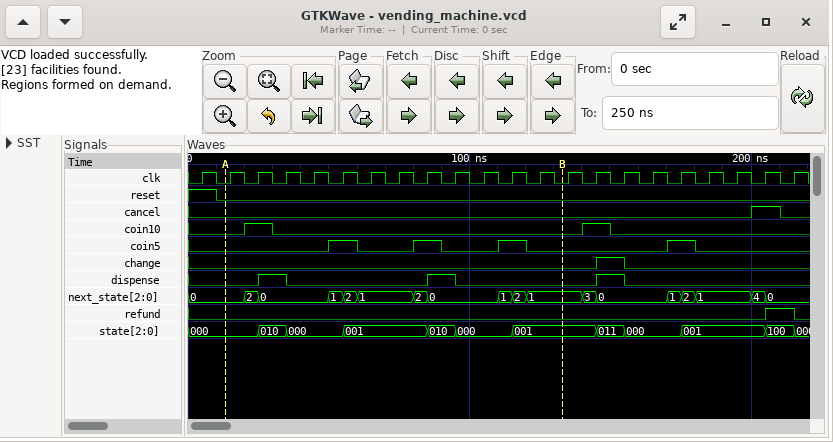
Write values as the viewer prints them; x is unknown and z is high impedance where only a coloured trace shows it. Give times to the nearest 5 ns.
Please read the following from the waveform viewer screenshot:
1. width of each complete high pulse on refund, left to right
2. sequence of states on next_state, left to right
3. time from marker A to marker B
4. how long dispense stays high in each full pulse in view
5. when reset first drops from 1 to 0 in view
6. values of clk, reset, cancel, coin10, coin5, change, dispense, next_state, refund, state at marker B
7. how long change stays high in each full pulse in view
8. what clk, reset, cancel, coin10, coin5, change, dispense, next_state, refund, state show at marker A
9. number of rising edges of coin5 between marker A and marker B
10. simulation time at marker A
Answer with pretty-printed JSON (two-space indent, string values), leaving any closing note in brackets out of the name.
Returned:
{
  "width of each complete high pulse on refund, left to right": "10 ns",
  "sequence of states on next_state, left to right": "0, 2, 0, 1, 2, 1, 2, 0, 1, 2, 1, 3, 0, 1, 2, 1, 4, 0",
  "time from marker A to marker B": "120 ns",
  "how long dispense stays high in each full pulse in view": "10 ns, 10 ns, 10 ns",
  "when reset first drops from 1 to 0 in view": "10 ns",
  "values of clk, reset, cancel, coin10, coin5, change, dispense, next_state, refund, state at marker B": "clk=0, reset=0, cancel=0, coin10=0, coin5=0, change=0, dispense=0, next_state=1, refund=0, state=001",
  "how long change stays high in each full pulse in view": "10 ns",
  "what clk, reset, cancel, coin10, coin5, change, dispense, next_state, refund, state show at marker A": "clk=0, reset=0, cancel=0, coin10=0, coin5=0, change=0, dispense=0, next_state=0, refund=0, state=000",
  "number of rising edges of coin5 between marker A and marker B": "3",
  "simulation time at marker A": "15 ns"
}
